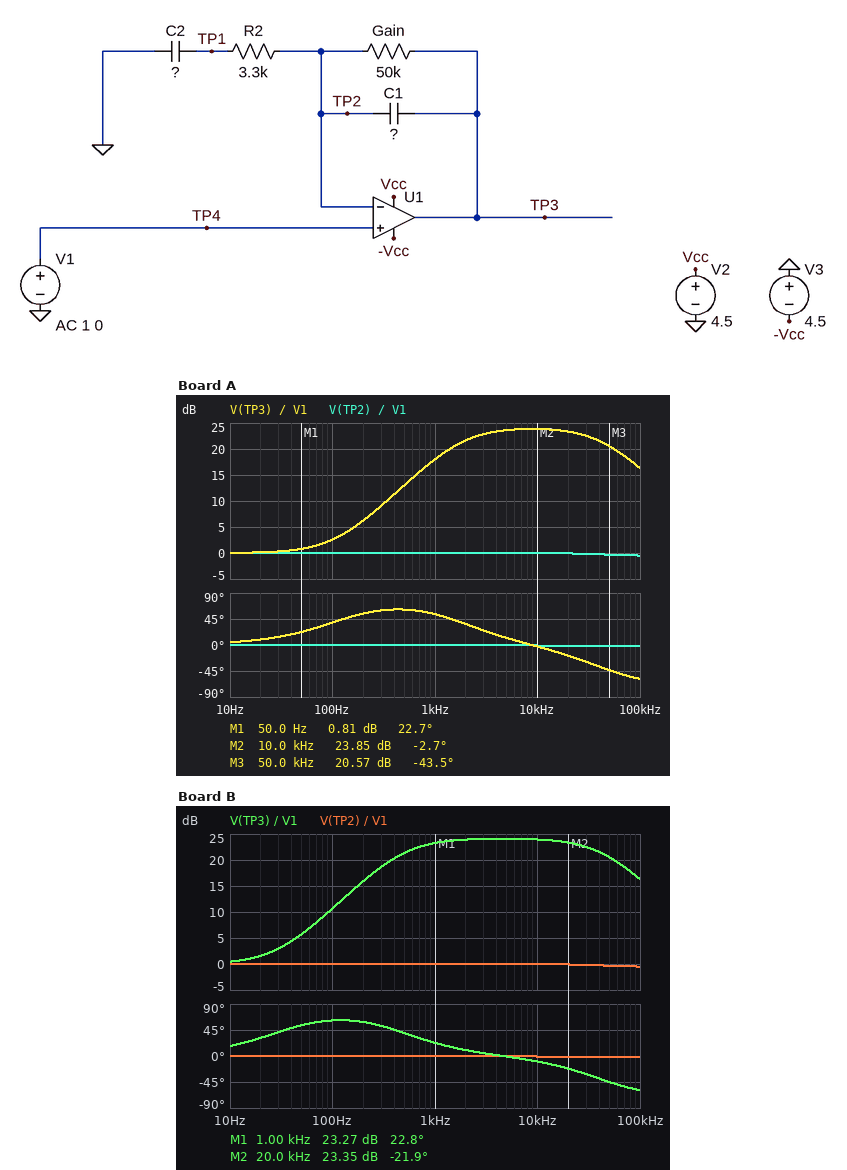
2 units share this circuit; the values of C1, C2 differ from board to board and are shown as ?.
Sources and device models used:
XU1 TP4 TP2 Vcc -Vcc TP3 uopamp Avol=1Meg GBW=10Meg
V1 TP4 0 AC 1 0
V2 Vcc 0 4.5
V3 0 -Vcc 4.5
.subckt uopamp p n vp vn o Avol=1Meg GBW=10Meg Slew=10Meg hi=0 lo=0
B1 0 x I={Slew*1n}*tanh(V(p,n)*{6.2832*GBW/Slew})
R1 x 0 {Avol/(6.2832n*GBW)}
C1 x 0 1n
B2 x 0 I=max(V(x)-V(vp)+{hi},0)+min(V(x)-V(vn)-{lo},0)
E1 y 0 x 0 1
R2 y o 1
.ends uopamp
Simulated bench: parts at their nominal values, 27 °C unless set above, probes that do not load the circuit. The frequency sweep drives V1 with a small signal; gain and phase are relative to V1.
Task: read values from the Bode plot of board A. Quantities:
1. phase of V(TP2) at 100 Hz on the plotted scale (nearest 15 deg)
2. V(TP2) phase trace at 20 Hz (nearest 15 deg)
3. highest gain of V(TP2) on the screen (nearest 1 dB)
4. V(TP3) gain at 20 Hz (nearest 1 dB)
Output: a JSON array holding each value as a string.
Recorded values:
["0 deg", "0 deg", "0 dB", "0 dB"]
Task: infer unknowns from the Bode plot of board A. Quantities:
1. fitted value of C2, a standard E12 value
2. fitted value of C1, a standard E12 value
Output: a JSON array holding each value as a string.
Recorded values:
["27 nF", "68 pF"]
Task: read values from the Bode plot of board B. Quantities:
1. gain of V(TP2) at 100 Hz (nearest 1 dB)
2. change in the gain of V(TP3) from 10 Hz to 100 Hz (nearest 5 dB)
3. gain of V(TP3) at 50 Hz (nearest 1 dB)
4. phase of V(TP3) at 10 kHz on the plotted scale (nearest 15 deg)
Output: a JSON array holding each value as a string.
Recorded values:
["0 dB", "10 dB", "6 dB", "-15 deg"]
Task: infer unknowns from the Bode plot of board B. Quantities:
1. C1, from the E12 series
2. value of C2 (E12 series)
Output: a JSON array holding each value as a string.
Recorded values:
["68 pF", "100 nF"]
